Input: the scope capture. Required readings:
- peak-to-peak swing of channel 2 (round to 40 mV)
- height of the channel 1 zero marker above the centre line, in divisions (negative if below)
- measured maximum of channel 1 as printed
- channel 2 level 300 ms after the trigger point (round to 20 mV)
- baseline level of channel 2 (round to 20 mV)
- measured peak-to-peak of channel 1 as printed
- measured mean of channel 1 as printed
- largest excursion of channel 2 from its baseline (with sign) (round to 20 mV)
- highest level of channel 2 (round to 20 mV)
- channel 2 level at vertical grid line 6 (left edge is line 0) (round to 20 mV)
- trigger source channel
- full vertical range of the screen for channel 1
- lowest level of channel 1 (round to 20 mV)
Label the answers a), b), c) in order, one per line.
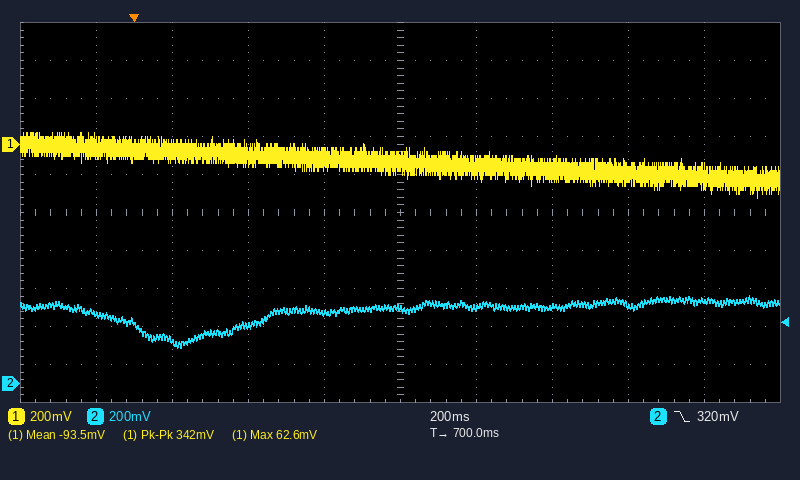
a) 280 mV
b) +1.8 div
c) 62.6 mV
d) 300 mV
e) 400 mV
f) 342 mV
g) -93.5 mV
h) -220 mV
i) 460 mV
j) 400 mV
k) channel 2
l) 2 V
m) -280 mV
